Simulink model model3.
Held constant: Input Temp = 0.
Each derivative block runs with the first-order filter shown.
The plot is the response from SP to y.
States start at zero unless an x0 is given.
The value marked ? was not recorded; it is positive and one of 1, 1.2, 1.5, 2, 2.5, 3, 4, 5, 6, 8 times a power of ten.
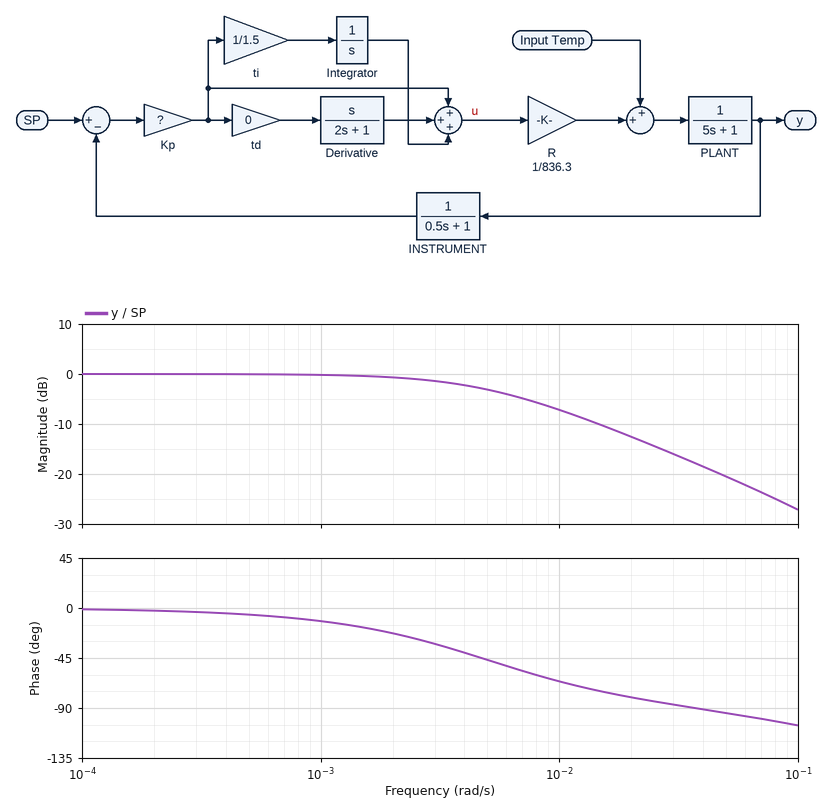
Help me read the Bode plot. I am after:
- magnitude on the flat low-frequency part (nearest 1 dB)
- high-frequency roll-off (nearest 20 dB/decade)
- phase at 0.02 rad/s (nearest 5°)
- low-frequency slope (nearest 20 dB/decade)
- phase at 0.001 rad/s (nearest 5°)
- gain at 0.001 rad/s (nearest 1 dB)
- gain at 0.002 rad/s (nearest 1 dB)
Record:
0 dB
-20 dB/decade
-80°
0 dB/decade
-10°
0 dB
-1 dB
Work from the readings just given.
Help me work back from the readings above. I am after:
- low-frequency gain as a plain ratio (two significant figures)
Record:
1.0
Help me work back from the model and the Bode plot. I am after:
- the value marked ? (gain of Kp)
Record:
6
